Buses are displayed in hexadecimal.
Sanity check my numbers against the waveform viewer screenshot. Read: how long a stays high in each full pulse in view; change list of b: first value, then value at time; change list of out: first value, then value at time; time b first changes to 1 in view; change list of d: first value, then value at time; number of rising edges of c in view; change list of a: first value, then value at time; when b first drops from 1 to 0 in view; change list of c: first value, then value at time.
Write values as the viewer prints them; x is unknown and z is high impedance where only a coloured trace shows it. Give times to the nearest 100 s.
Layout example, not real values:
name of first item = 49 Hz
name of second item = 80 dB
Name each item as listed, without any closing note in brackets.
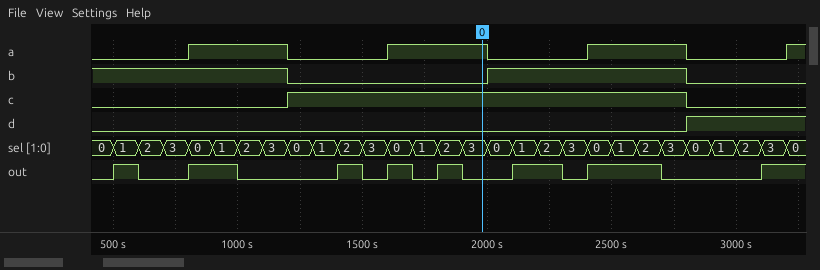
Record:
how long a stays high in each full pulse in view = 400 s, 400 s, 400 s
change list of b: first value, then value at time = 1, 0 at 1200 s, 1 at 2000 s, 0 at 2800 s
change list of out: first value, then value at time = 0, 1 at 500 s, 0 at 600 s, 1 at 800 s, 0 at 1000 s, 1 at 1400 s, 0 at 1500 s, 1 at 1600 s, 0 at 1700 s, 1 at 1800 s, 0 at 1900 s, 1 at 2100 s, 0 at 2300 s, 1 at 2400 s, 0 at 2700 s, 1 at 3100 s
time b first changes to 1 in view = 2000 s
change list of d: first value, then value at time = 0, 1 at 2800 s
number of rising edges of c in view = 1
change list of a: first value, then value at time = 0, 1 at 800 s, 0 at 1200 s, 1 at 1600 s, 0 at 2000 s, 1 at 2400 s, 0 at 2800 s, 1 at 3200 s
when b first drops from 1 to 0 in view = 1200 s
change list of c: first value, then value at time = 0, 1 at 1200 s, 0 at 2800 s
